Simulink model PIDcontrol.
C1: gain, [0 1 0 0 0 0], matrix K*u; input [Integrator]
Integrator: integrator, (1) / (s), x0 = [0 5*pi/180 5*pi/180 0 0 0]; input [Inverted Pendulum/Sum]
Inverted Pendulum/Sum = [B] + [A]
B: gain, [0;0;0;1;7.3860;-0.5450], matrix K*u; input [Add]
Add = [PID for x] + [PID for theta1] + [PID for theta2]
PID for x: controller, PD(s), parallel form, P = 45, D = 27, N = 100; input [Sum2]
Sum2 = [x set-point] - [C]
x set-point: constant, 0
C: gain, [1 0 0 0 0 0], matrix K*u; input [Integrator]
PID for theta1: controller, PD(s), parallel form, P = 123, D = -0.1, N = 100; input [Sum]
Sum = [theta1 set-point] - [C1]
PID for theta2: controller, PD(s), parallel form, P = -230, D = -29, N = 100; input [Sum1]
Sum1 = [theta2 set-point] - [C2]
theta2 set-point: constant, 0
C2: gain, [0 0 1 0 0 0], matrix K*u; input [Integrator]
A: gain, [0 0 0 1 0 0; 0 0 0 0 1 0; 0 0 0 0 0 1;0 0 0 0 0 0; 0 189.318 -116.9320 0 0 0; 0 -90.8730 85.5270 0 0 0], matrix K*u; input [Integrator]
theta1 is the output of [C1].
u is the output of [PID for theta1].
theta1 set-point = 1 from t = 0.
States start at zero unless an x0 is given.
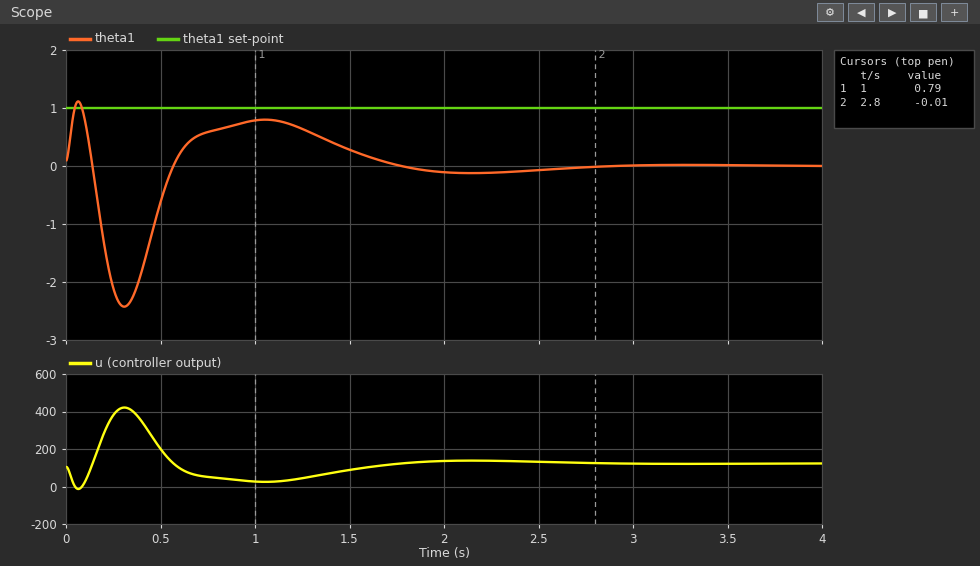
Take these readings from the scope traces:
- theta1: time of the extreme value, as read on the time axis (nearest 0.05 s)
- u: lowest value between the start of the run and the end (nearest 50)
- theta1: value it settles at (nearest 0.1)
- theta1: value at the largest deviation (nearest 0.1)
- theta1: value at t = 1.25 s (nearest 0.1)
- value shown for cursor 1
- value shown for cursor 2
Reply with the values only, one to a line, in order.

0.30 s
0
0.0
-2.4
0.6
0.79
-0.01
